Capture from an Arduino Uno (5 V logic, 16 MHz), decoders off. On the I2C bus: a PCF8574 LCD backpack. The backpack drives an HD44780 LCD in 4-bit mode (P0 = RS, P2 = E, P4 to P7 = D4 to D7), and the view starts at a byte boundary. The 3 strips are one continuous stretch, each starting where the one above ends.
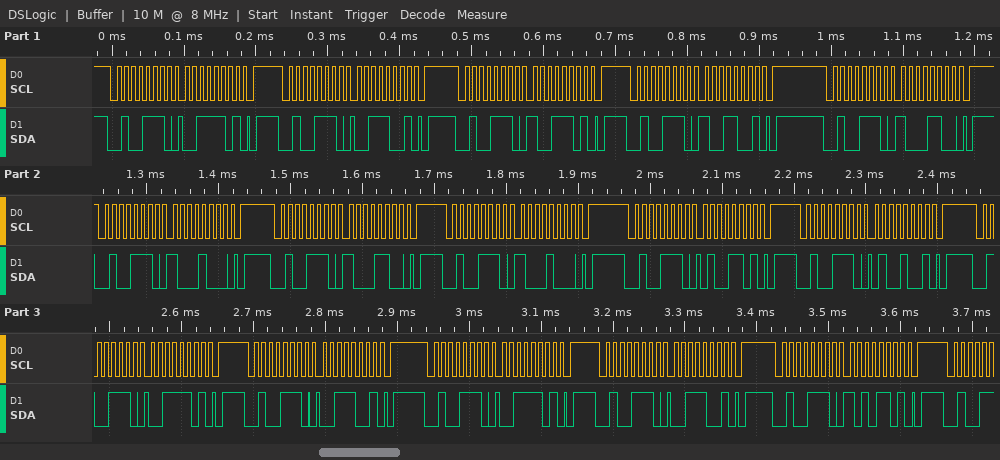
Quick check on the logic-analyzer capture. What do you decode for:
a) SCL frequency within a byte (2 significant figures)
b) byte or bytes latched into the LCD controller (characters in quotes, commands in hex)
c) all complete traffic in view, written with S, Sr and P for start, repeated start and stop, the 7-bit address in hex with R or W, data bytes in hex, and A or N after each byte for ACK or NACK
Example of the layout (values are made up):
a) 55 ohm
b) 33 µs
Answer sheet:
a) 100 kHz
b) '9' 0x88 'C'
c) S 27W A 3D A P S 27W A 39 A P S 27W A 9D A P S 27W A 99 A P S 27W A 8C A P S 27W A 88 A P S 27W A 8C A P S 27W A 88 A P S 27W A 4D A P S 27W A 49 A P S 27W A 3D A P S 27W A 39 A P S 27W A 3D A P S 27W A 39 A P S 27W A AD A P
